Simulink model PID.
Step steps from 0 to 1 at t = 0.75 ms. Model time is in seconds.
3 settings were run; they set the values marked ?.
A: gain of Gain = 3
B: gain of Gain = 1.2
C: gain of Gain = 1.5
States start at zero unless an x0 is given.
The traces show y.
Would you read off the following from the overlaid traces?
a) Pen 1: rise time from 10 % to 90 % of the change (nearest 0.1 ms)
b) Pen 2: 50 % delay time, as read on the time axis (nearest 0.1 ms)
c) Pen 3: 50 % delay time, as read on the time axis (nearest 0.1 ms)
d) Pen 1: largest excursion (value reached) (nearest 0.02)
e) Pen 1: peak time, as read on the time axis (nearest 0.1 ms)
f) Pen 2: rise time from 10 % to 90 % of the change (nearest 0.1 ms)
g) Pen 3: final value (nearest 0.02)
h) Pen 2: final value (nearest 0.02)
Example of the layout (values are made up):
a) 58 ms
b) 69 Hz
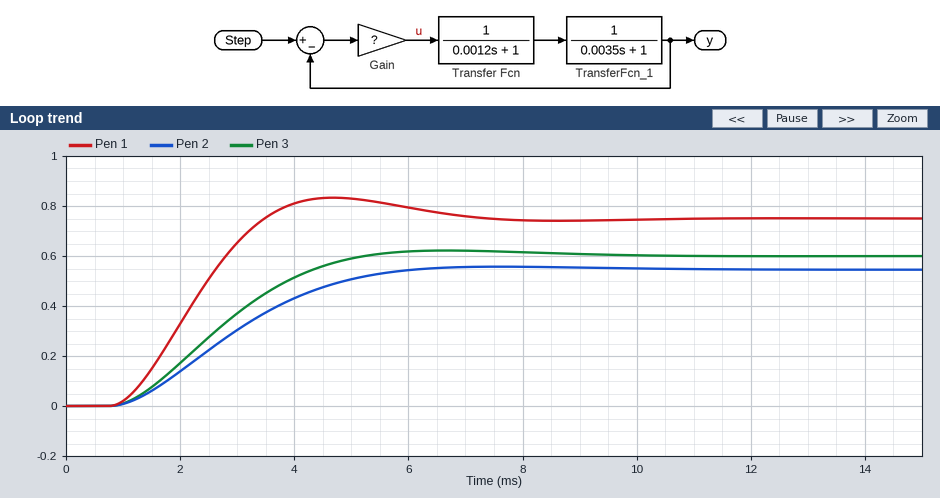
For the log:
a) 1.8 ms
b) 2.8 ms
c) 2.6 ms
d) 0.84
e) 4.7 ms
f) 3.3 ms
g) 0.60
h) 0.54
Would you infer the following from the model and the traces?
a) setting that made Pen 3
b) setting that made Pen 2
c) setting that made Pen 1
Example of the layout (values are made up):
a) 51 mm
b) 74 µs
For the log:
a) C
b) B
c) A
